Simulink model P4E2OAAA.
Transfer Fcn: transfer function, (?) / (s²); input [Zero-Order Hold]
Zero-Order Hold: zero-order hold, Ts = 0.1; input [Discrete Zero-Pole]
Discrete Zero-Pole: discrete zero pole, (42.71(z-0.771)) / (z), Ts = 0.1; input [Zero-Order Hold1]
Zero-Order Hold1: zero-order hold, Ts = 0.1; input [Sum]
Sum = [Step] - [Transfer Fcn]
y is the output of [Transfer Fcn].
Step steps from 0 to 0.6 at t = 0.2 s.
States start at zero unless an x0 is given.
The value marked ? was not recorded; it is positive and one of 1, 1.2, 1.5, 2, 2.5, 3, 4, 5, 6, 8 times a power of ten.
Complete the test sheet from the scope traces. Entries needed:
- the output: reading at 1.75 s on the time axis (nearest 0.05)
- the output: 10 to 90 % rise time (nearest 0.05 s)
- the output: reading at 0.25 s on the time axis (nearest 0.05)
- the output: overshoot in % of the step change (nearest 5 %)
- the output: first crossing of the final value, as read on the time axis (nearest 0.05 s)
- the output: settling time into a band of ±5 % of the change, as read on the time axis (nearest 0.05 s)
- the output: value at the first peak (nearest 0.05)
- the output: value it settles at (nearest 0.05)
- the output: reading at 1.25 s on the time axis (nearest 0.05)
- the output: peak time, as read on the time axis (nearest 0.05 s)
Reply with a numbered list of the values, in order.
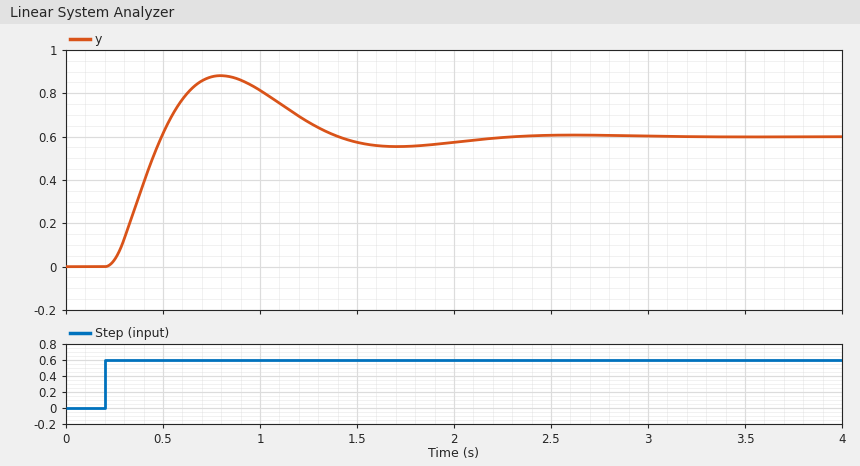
1. 0.55
2. 0.20 s
3. 0.05
4. 45 %
5. 0.50 s
6. 1.95 s
7. 0.90
8. 0.60
9. 0.65
10. 0.80 s
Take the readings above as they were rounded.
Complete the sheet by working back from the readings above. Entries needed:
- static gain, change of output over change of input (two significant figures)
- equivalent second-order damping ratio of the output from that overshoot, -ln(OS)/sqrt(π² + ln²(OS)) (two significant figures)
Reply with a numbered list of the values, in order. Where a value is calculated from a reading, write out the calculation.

1. (0.6 - 0) / (0.6 - 0) = 1.0
2. ln(0.45) = -0.799; 0.799 / sqrt(9.870 + 0.638) = 0.25
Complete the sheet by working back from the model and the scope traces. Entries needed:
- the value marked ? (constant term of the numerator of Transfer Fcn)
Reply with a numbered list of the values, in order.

1. 1
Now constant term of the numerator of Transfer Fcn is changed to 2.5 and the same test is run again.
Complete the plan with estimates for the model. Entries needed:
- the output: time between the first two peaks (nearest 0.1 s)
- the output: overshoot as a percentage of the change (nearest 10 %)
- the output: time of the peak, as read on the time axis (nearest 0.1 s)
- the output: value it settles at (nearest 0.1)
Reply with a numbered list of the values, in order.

1. 0.6 s
2. 80 %
3. 0.5 s
4. 0.6
